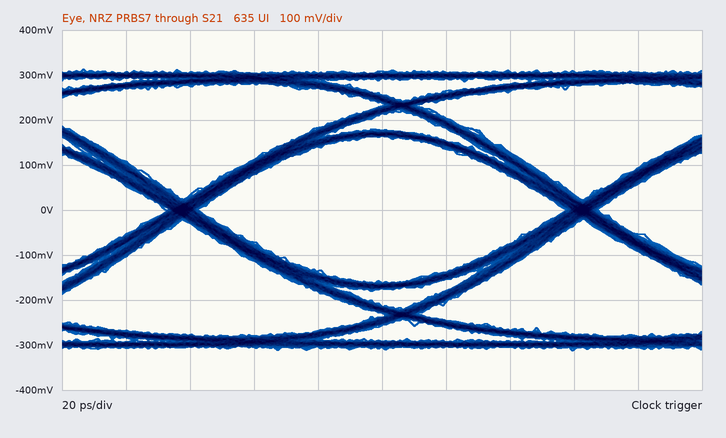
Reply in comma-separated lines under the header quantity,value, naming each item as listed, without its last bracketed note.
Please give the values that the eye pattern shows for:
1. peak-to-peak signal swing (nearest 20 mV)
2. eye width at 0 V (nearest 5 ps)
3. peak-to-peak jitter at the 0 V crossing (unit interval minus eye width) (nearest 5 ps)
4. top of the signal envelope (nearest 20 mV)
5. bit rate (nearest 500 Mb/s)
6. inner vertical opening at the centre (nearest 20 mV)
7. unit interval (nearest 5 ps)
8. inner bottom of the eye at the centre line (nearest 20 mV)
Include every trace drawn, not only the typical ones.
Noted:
quantity,value
peak-to-peak signal swing,620 mV
eye width at 0 V,115 ps
peak-to-peak jitter at the 0 V crossing (unit interval minus eye width),10 ps
top of the signal envelope,320 mV
bit rate,8.0 Gb/s
inner vertical opening at the centre,320 mV
unit interval,125 ps
inner bottom of the eye at the centre line,-160 mV
